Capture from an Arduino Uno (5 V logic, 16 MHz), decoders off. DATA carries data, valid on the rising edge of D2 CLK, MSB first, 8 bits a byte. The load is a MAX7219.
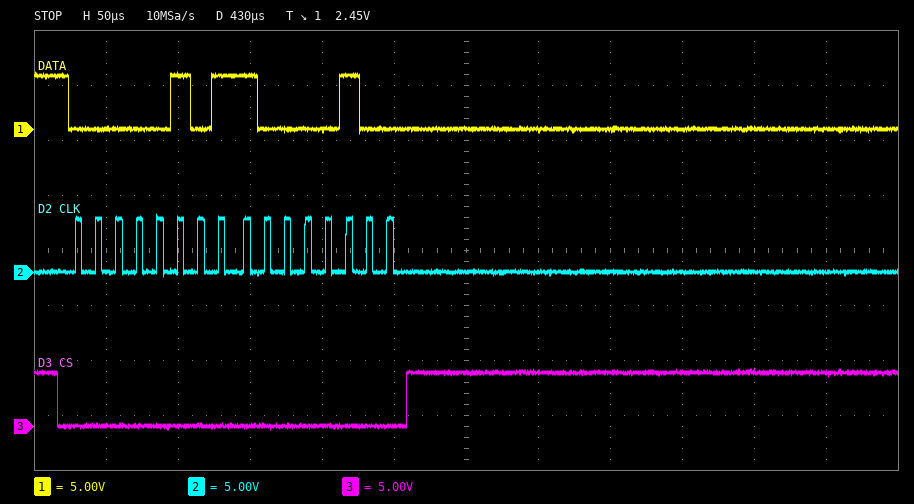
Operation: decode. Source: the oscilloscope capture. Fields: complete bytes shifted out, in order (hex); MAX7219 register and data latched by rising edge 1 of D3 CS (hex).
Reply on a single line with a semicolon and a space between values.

05 84; register 0x5, data 0x84
